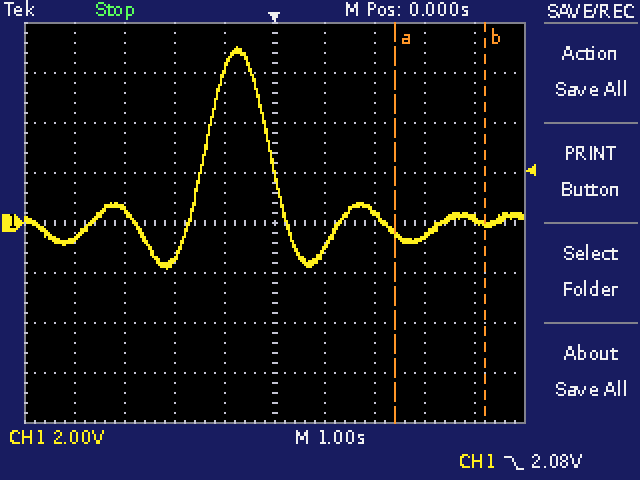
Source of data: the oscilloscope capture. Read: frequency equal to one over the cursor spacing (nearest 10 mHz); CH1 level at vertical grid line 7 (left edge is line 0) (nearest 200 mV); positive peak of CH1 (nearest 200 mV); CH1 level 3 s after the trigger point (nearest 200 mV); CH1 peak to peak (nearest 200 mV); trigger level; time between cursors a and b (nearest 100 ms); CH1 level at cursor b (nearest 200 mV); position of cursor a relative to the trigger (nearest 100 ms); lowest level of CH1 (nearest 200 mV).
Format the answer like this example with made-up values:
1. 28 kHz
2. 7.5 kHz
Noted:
1. 560 mHz
2. 400 mV
3. 7.0 V
4. -600 mV
5. 8.8 V
6. 2.08 V
7. 1.8 s
8. 0.0 V
9. +2.4 s
10. -1.8 V
